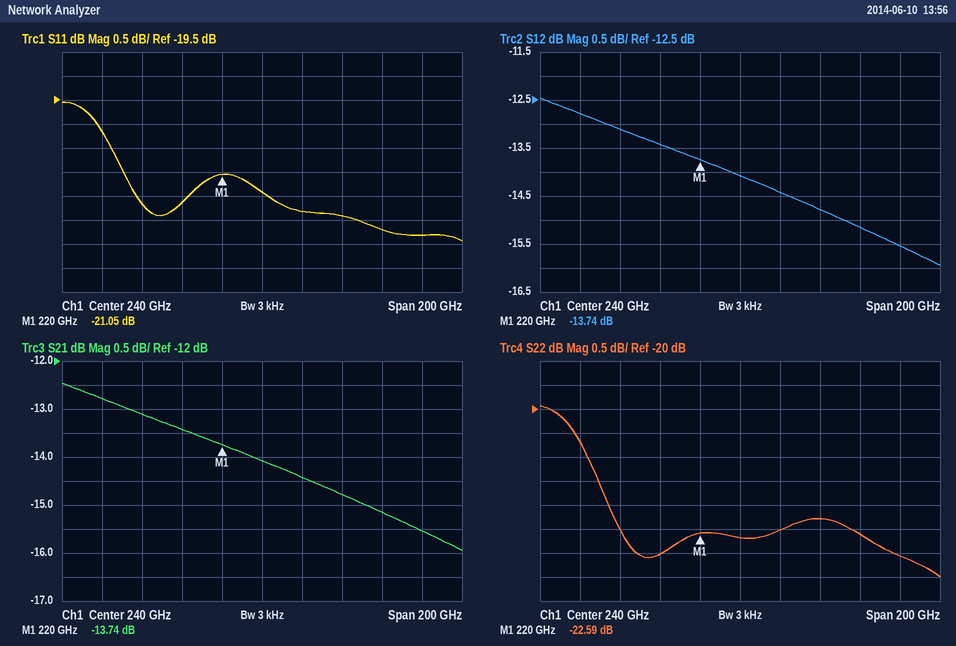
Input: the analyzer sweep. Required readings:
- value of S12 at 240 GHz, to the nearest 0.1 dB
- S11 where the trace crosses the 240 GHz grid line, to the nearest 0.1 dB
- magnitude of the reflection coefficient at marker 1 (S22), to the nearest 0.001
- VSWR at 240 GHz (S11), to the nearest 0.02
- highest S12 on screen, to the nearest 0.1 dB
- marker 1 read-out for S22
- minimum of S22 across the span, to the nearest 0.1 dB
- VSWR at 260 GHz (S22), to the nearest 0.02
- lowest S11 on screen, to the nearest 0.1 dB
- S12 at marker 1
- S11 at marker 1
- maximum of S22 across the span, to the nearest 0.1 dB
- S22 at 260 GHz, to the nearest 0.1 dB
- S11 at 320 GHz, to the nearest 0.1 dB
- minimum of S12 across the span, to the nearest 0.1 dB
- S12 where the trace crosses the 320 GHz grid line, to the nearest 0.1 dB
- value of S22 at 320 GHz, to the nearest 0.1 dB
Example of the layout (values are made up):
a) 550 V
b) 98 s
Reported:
a) -14.1 dB
b) -21.4 dB
c) 0.074
d) 1.18
e) -12.5 dB
f) -22.59 dB
g) -23.5 dB
h) 1.16
i) -22.4 dB
j) -13.74 dB
k) -21.05 dB
l) -19.9 dB
m) -22.5 dB
n) -22.3 dB
o) -15.9 dB
p) -15.5 dB
q) -23.1 dB
